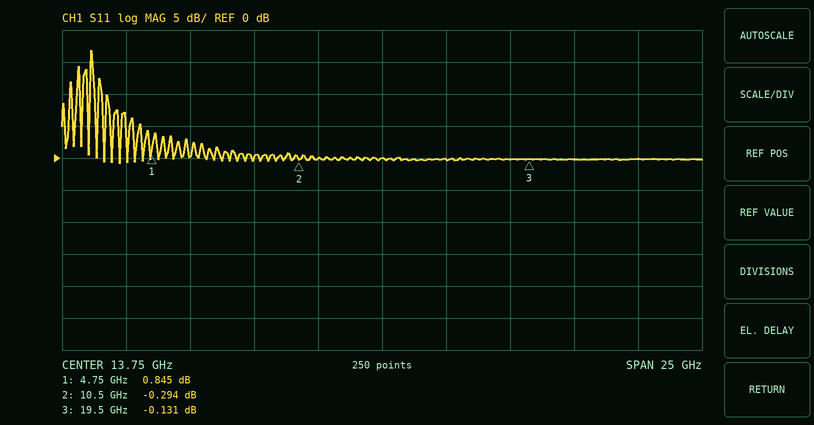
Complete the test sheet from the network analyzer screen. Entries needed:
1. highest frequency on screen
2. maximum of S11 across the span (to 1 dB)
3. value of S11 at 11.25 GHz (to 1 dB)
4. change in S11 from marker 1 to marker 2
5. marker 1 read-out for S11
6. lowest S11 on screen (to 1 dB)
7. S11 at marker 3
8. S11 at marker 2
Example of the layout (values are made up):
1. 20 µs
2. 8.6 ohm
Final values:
1. 26.25 GHz
2. 17 dB
3. 0 dB
4. -1.139 dB
5. 0.845 dB
6. -1 dB
7. -0.131 dB
8. -0.294 dB
